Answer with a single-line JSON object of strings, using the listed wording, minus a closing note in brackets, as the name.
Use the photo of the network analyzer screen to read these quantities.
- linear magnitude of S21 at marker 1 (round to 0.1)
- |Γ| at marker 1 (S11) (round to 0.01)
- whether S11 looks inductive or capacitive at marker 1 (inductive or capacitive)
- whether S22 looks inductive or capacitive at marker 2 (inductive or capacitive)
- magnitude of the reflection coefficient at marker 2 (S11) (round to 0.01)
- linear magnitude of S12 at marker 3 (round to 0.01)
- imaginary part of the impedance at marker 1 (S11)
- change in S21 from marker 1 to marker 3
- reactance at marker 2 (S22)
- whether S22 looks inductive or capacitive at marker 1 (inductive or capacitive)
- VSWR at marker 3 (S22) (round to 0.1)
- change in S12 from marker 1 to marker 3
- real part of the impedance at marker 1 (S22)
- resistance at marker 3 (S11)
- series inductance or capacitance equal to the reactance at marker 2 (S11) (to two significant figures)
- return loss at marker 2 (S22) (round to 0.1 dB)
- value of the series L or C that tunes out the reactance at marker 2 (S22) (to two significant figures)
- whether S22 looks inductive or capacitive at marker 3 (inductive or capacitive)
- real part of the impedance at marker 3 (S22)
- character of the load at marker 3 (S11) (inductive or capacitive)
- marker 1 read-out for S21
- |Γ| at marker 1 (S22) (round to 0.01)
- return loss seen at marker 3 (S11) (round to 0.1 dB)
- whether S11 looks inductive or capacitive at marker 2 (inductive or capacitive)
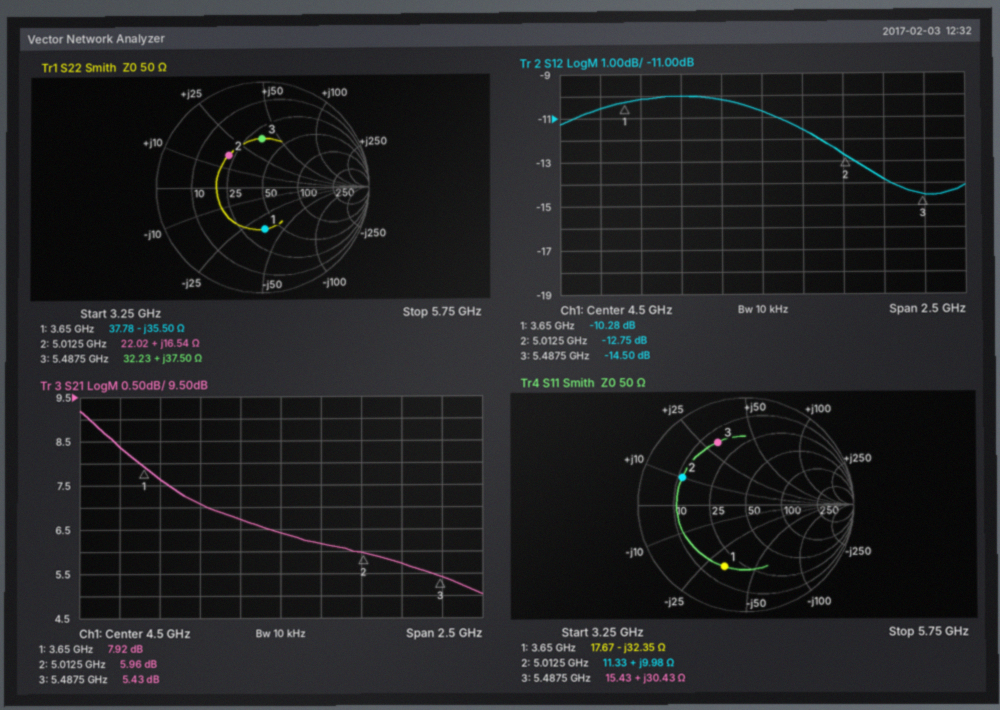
{"linear magnitude of S21 at marker 1": "2.5", "|Γ| at marker 1 (S11)": "0.61", "whether S11 looks inductive or capacitive at marker 1": "capacitive", "whether S22 looks inductive or capacitive at marker 2": "inductive", "magnitude of the reflection coefficient at marker 2 (S11)": "0.64", "linear magnitude of S12 at marker 3": "0.19", "imaginary part of the impedance at marker 1": "-32.35 Ω", "change in S21 from marker 1 to marker 3": "-2.49 dB", "reactance at marker 2": "+16.54 Ω", "whether S22 looks inductive or capacitive at marker 1": "capacitive", "VSWR at marker 3 (S22)": "2.7", "change in S12 from marker 1 to marker 3": "-4.22 dB", "real part of the impedance at marker 1": "37.78 Ω", "resistance at marker 3": "15.43 Ω", "series inductance or capacitance equal to the reactance at marker 2 (S11)": "320 pH", "return loss at marker 2 (S22)": "7.1 dB", "value of the series L or C that tunes out the reactance at marker 2 (S22)": "1.9 pF", "whether S22 looks inductive or capacitive at marker 3": "inductive", "real part of the impedance at marker 3": "32.23 Ω", "character of the load at marker 3 (S11)": "inductive", "marker 1 read-out for S21": "7.92 dB", "|Γ| at marker 1 (S22)": "0.40", "return loss seen at marker 3 (S11)": "3.9 dB", "whether S11 looks inductive or capacitive at marker 2": "inductive"}
